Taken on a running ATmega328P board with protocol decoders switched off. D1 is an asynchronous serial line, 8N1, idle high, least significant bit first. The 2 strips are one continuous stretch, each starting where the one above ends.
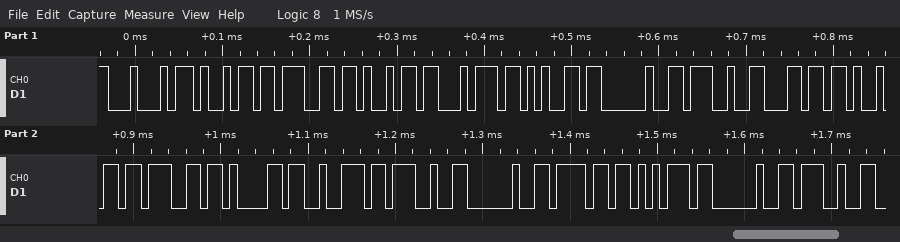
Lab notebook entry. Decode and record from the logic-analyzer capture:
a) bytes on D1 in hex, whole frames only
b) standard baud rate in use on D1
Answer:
44 69 67 69 74 65 20 27 6C 69 67 61 72 27 20 6F 75 20 27
115200 baud
